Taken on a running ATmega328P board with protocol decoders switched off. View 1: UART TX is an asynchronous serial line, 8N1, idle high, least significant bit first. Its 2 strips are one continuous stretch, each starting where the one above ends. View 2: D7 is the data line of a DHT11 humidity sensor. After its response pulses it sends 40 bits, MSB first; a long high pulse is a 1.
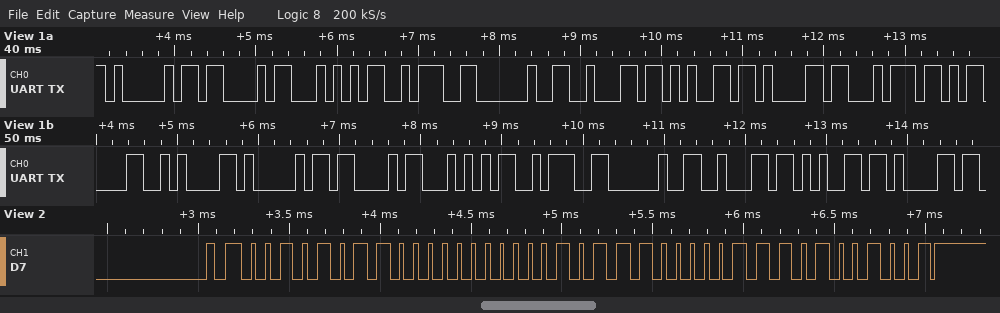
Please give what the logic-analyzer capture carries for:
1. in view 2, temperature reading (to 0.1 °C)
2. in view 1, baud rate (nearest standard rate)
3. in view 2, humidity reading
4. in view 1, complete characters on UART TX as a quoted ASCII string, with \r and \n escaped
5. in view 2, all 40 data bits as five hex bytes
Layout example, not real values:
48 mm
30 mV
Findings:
23.7 °C
9600 baud
43 %
"ACT: beat\r\nACT: bea"
2B 00 17 07 49
